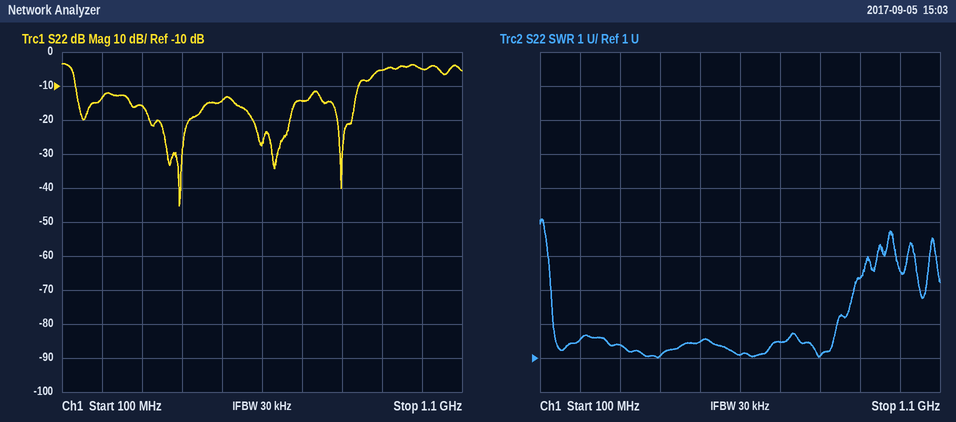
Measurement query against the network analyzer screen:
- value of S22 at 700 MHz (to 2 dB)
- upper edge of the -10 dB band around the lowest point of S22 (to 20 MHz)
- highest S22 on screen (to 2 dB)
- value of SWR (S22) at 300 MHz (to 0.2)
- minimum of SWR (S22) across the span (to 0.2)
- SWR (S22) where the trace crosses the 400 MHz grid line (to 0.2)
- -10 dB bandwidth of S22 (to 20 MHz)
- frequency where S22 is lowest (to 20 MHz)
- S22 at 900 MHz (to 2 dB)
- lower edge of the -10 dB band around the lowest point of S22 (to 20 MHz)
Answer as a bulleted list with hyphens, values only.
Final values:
- -14 dB
- 840 MHz
- -4 dB
- 1.4
- 1.0
- 1.0
- 700 MHz
- 400 MHz
- -6 dB
- 140 MHz
